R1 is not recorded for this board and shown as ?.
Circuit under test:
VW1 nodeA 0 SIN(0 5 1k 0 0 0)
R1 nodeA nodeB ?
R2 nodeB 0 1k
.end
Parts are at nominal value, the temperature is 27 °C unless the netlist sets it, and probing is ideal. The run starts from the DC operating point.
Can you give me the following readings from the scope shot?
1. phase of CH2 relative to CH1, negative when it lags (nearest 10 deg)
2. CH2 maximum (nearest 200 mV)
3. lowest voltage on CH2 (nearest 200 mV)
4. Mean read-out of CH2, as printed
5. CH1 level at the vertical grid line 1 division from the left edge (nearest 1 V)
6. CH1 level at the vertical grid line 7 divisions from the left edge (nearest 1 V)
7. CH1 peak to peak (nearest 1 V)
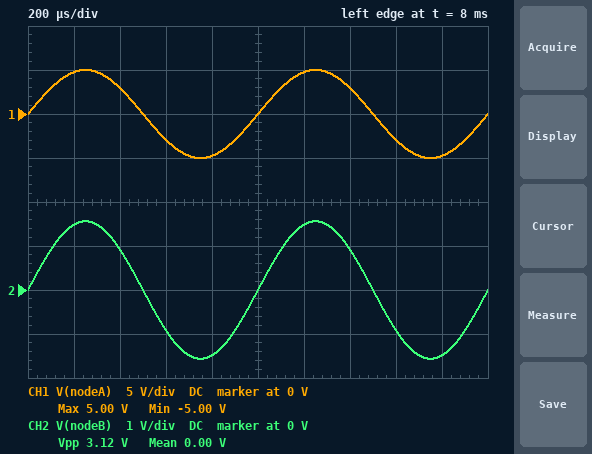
0 deg
1.6 V
-1.6 V
0.00 V
5 V
3 V
10 V
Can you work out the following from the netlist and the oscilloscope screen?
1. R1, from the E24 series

2.2 kΩ
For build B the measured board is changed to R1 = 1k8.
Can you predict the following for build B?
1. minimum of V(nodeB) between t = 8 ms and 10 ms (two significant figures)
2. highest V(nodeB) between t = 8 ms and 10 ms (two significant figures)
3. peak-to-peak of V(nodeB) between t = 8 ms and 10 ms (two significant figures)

-1.8 V
1.8 V
3.6 V
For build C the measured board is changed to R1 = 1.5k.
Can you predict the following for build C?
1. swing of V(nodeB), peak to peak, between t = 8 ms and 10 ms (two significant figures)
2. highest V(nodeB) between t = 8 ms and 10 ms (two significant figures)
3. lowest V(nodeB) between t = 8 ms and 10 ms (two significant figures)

4.0 V
2.0 V
-2.0 V
